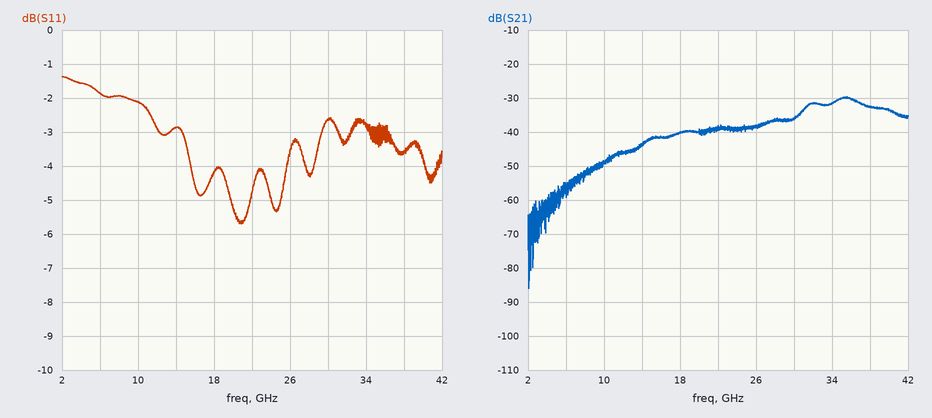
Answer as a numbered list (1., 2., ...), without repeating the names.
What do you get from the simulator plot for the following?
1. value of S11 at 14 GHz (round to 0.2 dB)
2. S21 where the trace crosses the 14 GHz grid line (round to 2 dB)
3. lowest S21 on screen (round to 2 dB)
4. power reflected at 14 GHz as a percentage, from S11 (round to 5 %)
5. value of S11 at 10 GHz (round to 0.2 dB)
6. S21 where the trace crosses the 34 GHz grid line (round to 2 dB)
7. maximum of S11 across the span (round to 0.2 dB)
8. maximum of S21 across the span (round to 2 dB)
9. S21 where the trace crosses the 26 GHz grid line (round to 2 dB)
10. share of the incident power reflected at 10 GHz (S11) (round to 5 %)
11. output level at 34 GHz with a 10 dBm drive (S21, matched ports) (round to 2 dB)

1. -2.8 dB
2. -44 dB
3. -86 dB
4. 50 %
5. -2.2 dB
6. -32 dB
7. -1.4 dB
8. -30 dB
9. -38 dB
10. 60 %
11. -22 dBm
